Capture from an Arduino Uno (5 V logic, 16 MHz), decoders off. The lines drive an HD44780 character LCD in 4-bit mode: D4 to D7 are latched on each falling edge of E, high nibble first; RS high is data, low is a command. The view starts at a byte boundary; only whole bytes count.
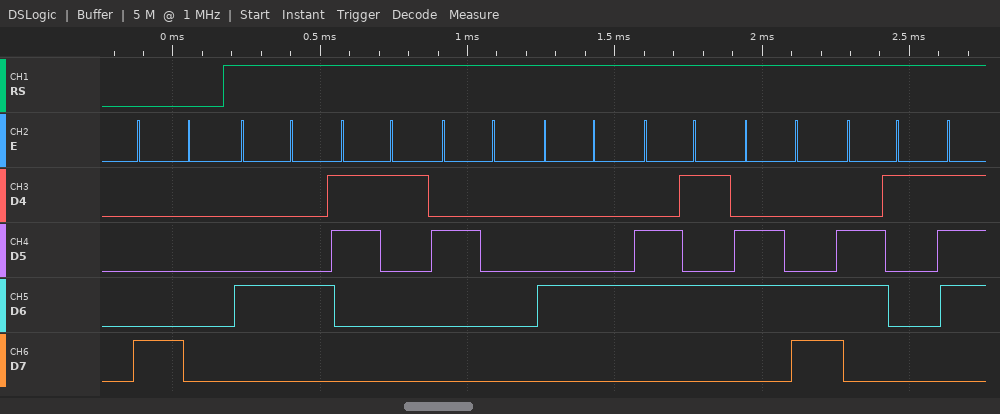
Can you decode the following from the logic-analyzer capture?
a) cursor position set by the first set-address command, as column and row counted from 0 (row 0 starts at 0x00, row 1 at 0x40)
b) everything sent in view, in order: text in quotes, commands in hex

column 0, row 0
0x80 "D1 Dela"
